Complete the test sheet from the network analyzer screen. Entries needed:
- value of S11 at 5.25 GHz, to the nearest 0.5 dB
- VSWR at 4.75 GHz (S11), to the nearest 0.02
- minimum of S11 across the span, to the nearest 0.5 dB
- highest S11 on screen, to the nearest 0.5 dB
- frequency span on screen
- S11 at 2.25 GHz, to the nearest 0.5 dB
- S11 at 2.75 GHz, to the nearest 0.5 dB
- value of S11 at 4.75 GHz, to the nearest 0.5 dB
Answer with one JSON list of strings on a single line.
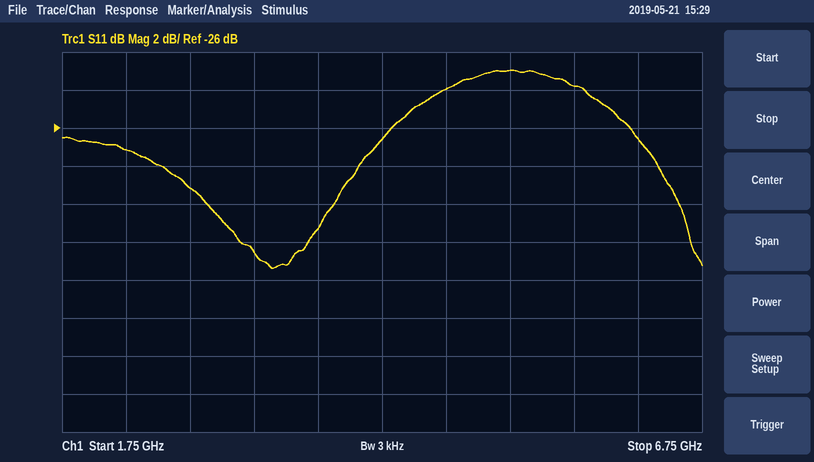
["-23.0 dB", "1.14", "-33.5 dB", "-23.0 dB", "5 GHz", "-27.0 dB", "-29.0 dB", "-24.0 dB"]
